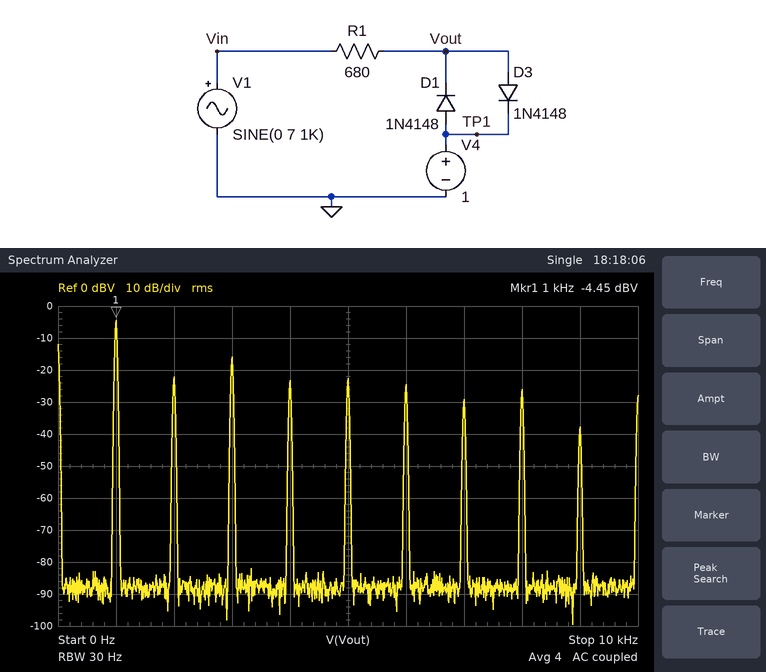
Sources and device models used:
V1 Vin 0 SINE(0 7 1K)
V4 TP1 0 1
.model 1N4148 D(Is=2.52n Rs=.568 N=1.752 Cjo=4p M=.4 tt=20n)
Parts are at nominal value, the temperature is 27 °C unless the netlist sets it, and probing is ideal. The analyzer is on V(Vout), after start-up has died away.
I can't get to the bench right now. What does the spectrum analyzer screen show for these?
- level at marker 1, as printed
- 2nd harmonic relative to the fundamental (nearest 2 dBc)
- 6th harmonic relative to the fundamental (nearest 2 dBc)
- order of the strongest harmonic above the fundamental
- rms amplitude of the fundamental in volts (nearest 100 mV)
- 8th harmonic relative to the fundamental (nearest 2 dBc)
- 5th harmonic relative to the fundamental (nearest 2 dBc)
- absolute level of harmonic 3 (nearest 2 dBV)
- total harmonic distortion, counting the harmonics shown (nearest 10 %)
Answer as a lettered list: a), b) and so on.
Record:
a) -4.45 dBV
b) -18 dBc
c) -20 dBc
d) 3
e) 600 mV
f) -22 dBc
g) -18 dBc
h) -16 dBV
i) 40 %
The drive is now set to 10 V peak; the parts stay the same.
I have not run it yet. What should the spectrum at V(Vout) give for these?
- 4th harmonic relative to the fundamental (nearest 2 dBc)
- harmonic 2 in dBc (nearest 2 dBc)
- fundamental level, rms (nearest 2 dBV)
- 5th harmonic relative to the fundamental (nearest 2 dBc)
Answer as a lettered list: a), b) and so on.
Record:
a) -22 dBc
b) -20 dBc
c) -4 dBV
d) -16 dBc
